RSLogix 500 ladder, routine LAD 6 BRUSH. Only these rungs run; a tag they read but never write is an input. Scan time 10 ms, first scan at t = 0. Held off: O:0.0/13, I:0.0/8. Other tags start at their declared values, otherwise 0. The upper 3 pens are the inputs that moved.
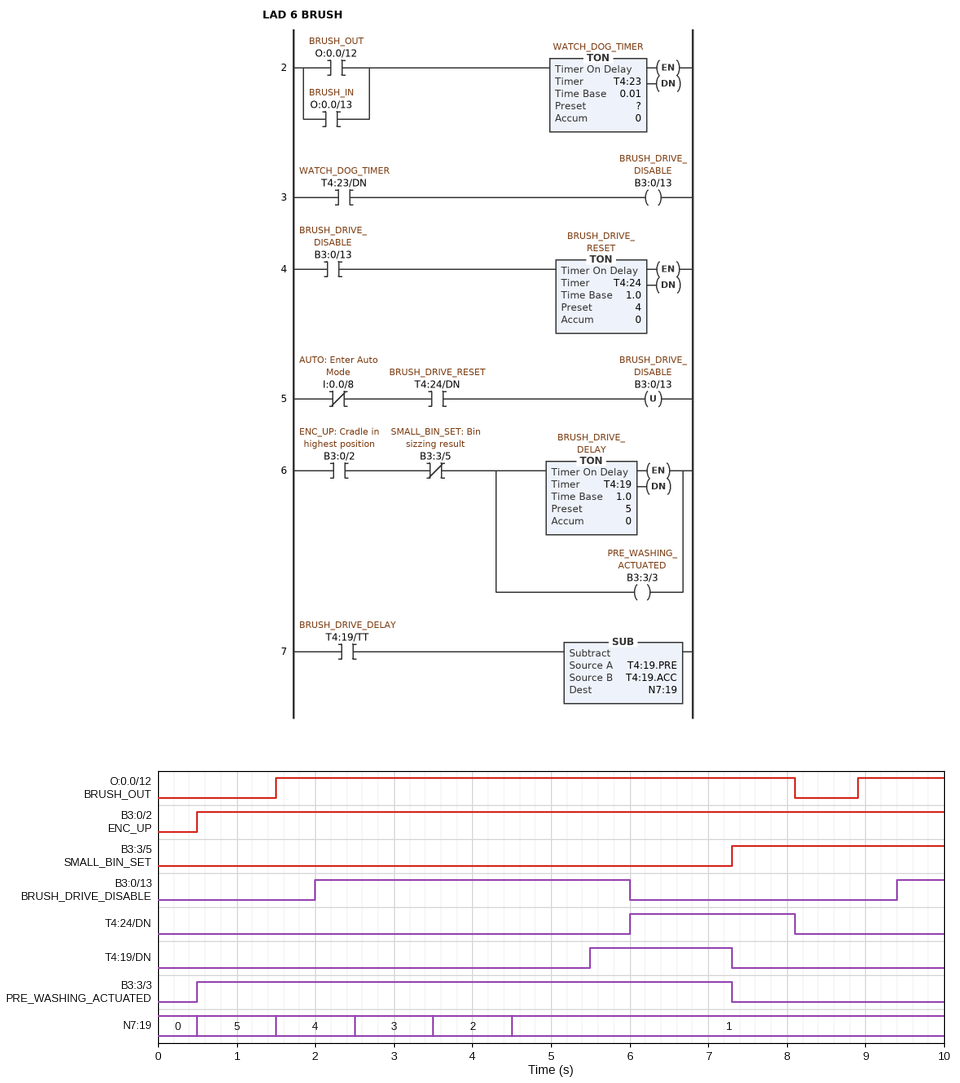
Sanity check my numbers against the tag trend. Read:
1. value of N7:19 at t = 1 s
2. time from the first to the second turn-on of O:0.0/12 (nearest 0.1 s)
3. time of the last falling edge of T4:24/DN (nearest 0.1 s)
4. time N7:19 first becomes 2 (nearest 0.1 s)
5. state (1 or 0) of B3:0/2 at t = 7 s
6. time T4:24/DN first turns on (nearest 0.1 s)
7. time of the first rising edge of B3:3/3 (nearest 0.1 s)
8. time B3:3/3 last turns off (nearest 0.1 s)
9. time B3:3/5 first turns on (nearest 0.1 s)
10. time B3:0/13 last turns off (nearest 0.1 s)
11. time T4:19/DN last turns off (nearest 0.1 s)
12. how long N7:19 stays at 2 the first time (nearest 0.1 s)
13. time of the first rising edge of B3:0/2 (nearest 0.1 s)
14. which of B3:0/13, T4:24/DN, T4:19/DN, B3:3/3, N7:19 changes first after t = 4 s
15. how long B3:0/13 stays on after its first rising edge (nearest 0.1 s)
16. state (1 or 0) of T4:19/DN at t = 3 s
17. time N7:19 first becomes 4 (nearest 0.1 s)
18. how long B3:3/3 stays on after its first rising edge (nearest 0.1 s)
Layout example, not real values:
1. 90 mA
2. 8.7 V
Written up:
1. 5
2. 7.4 s
3. 8.1 s
4. 3.5 s
5. 1
6. 6.0 s
7. 0.5 s
8. 7.3 s
9. 7.3 s
10. 6.0 s
11. 7.3 s
12. 1.0 s
13. 0.5 s
14. N7:19
15. 4.0 s
16. 0
17. 1.5 s
18. 6.8 s
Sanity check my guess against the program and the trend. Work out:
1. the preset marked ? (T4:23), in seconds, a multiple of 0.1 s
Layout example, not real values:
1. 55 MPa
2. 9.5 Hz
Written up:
1. 0.5 s
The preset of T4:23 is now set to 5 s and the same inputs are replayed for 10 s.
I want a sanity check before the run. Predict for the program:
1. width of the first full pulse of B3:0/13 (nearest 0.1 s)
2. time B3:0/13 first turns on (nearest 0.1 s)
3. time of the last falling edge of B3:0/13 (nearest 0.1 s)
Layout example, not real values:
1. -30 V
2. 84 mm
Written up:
1. 1.6 s
2. 6.5 s
3. 8.1 s
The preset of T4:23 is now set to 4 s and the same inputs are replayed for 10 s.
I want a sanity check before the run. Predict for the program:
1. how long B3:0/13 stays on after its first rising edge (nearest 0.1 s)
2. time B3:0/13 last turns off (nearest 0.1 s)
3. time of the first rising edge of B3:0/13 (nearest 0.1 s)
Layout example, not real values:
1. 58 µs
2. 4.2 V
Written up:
1. 2.6 s
2. 8.1 s
3. 5.5 s
